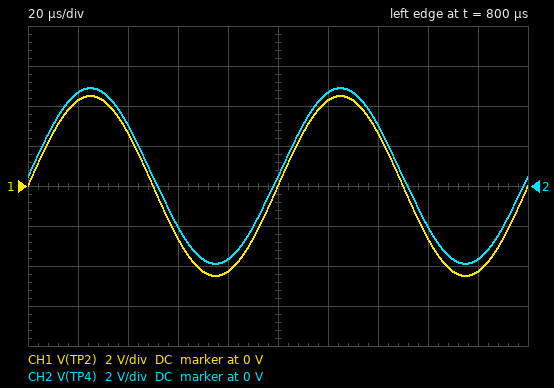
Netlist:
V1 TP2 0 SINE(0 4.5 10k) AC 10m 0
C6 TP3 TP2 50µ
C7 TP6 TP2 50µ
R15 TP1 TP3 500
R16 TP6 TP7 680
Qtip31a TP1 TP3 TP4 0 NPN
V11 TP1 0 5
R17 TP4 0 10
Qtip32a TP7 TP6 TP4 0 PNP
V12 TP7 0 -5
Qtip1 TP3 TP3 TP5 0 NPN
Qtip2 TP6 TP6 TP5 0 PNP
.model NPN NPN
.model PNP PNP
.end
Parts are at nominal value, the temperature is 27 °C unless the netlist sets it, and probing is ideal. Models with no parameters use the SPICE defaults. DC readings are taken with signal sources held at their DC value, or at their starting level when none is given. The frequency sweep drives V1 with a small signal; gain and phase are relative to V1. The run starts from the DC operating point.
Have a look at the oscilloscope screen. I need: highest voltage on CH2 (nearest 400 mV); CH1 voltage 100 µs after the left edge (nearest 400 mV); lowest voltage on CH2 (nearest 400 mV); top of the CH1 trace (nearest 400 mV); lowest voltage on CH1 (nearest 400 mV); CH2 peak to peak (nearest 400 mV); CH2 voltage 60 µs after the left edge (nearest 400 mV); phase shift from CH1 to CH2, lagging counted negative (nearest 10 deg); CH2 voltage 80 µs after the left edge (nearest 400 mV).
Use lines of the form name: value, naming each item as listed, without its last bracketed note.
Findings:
highest voltage on CH2: 4.8 V
CH1 voltage 100 µs after the left edge: 0 V
lowest voltage on CH2: -4.0 V
top of the CH1 trace: 4.4 V
lowest voltage on CH1: -4.4 V
CH2 peak to peak: 8.8 V
CH2 voltage 60 µs after the left edge: -2.0 V
phase shift from CH1 to CH2, lagging counted negative: 0 deg
CH2 voltage 80 µs after the left edge: -3.6 V
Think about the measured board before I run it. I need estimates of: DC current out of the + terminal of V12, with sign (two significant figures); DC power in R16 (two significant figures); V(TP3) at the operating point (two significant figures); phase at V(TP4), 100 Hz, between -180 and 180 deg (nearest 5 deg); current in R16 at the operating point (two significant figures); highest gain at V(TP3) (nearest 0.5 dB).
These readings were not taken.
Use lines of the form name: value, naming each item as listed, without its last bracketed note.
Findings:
DC current out of the + terminal of V12, with sign: -7.9 mA
DC power in R16: 32 mW
V(TP3) at the operating point: 1.3 V
phase at V(TP4), 100 Hz, between -180 and 180 deg: 5 deg
current in R16 at the operating point: 6.9 mA
highest gain at V(TP3): 0 dB
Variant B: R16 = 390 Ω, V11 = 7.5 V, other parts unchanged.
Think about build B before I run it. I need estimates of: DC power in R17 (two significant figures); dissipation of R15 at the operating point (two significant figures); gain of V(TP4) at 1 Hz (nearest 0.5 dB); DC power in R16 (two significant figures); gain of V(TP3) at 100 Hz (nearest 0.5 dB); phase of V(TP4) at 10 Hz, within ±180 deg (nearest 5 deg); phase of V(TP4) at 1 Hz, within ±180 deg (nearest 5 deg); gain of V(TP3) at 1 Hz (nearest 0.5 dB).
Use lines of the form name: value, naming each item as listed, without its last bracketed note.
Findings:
DC power in R17: 20 mW
dissipation of R15 at the operating point: 76 mW
gain of V(TP4) at 1 Hz: -19.5 dB
DC power in R16: 55 mW
gain of V(TP3) at 100 Hz: 0 dB
phase of V(TP4) at 10 Hz, within ±180 deg: 40 deg
phase of V(TP4) at 1 Hz, within ±180 deg: 85 deg
gain of V(TP3) at 1 Hz: -19.0 dB
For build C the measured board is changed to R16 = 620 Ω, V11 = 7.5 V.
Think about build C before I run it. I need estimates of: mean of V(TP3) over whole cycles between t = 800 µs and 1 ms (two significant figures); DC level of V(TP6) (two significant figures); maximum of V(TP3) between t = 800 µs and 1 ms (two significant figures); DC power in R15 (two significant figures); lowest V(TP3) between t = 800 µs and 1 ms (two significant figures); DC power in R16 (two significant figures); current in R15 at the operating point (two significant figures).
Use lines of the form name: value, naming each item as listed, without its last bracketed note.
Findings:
mean of V(TP3) over whole cycles between t = 800 µs and 1 ms: 2.3 V
DC level of V(TP6): 620 mV
maximum of V(TP3) between t = 800 µs and 1 ms: 6.8 V
DC power in R15: 54 mW
lowest V(TP3) between t = 800 µs and 1 ms: -2.2 V
DC power in R16: 51 mW
current in R15 at the operating point: 10 mA
